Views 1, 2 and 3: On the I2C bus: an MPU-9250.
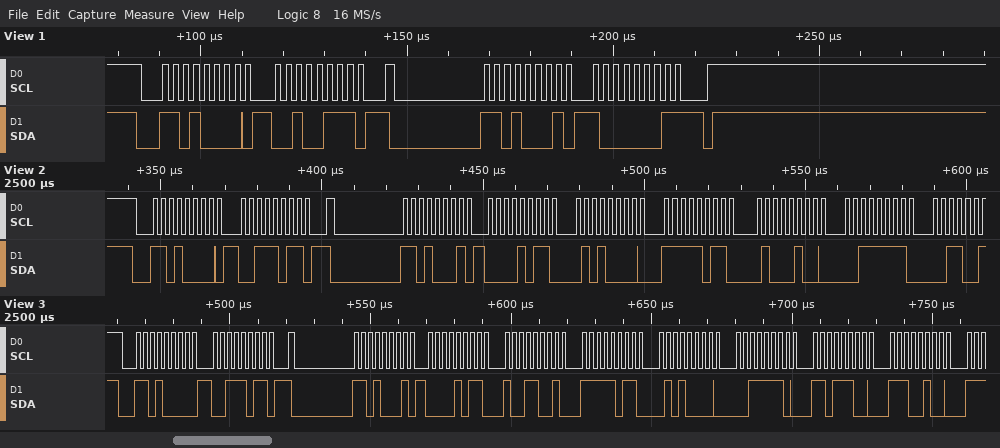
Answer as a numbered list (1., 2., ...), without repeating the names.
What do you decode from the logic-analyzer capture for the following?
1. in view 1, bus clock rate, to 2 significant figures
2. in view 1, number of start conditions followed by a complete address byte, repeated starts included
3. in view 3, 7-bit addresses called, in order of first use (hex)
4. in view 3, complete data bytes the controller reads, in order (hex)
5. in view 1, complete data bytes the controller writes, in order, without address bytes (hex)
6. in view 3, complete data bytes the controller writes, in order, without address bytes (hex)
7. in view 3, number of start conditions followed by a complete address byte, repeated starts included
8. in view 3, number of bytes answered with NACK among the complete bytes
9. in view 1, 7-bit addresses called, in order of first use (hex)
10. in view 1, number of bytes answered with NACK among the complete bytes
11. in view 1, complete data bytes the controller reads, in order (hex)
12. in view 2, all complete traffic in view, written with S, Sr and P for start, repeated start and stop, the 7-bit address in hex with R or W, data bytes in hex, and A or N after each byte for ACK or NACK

1. 400 kHz
2. 2
3. 0x68
4. 0B 99 FB 50 3E DC E4
5. 27
6. 3B
7. 2
8. 0
9. 0x68
10. 1
11. 81
12. S 68W A 3B A Sr 68R A 0B A 50 A FB A 44 A 3F A
